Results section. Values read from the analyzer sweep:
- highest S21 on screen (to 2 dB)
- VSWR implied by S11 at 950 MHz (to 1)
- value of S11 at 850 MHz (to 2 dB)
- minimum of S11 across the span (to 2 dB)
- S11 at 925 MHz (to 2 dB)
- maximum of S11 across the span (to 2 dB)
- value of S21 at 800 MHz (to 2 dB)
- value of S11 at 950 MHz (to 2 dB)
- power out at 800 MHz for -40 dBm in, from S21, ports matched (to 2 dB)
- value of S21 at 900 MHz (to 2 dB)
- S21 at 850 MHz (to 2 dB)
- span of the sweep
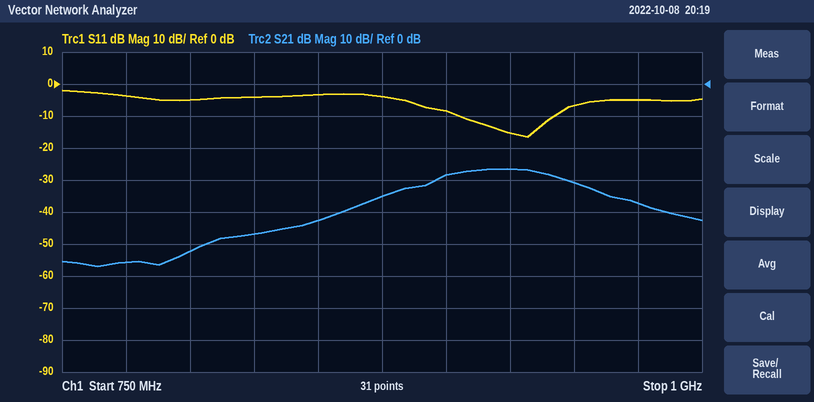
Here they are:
-26 dB
3
-4 dB
-16 dB
-16 dB
-2 dB
-52 dB
-6 dB
-92 dBm
-28 dB
-42 dB
250 MHz
